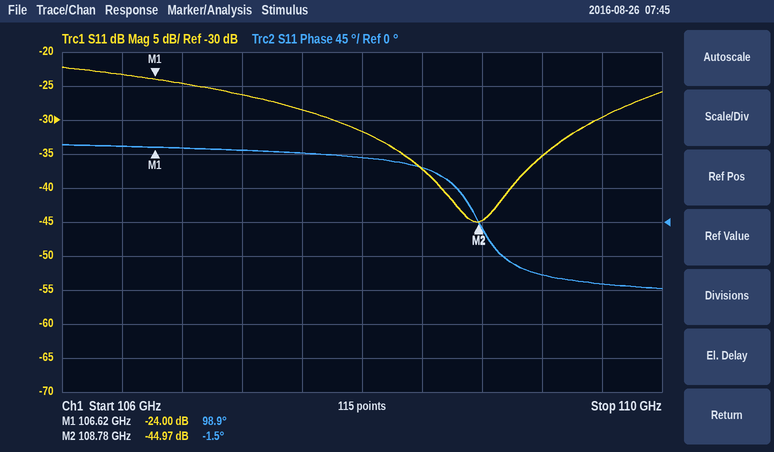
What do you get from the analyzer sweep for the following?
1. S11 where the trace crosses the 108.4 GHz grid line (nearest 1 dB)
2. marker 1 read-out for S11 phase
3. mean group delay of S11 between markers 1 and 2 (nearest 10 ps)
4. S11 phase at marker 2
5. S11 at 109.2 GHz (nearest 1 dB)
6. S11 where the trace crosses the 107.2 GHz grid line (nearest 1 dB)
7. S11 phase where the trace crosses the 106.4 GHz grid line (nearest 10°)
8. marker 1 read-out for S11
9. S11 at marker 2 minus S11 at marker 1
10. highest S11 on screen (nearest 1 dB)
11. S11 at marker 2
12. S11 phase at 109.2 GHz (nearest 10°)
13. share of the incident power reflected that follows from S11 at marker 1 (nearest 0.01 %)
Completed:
-37 dB
98.9°
130 ps
-1.5°
-35 dB
-26 dB
100°
-24.00 dB
-20.97 dB
-22 dB
-44.97 dB
-70°
0.40 %
